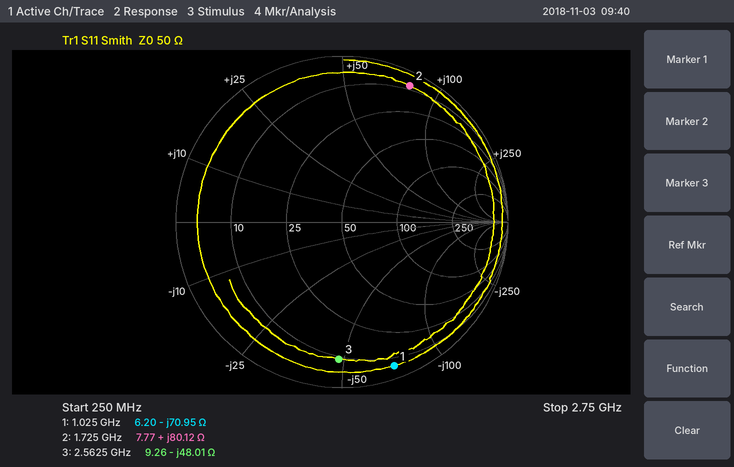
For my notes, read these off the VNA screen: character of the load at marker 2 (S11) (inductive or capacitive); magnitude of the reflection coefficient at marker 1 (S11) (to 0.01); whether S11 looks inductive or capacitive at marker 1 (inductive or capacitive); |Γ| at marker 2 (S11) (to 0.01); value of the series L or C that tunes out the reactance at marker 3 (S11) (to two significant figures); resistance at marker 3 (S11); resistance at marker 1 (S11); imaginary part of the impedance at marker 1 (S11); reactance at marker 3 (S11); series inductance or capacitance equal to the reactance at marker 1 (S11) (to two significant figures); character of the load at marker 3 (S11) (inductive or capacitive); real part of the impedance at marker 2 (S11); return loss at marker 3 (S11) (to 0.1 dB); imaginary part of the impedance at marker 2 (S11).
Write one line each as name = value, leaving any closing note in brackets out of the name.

character of the load at marker 2 (S11) = inductive
magnitude of the reflection coefficient at marker 1 (S11) = 0.92
whether S11 looks inductive or capacitive at marker 1 = capacitive
|Γ| at marker 2 (S11) = 0.92
value of the series L or C that tunes out the reactance at marker 3 (S11) = 3.0 nH
resistance at marker 3 = 9.26 Ω
resistance at marker 1 = 6.20 Ω
imaginary part of the impedance at marker 1 = -70.95 Ω
reactance at marker 3 = -48.01 Ω
series inductance or capacitance equal to the reactance at marker 1 (S11) = 2.2 pF
character of the load at marker 3 (S11) = capacitive
real part of the impedance at marker 2 = 7.77 Ω
return loss at marker 3 (S11) = 1.7 dB
imaginary part of the impedance at marker 2 = +80.12 Ω
